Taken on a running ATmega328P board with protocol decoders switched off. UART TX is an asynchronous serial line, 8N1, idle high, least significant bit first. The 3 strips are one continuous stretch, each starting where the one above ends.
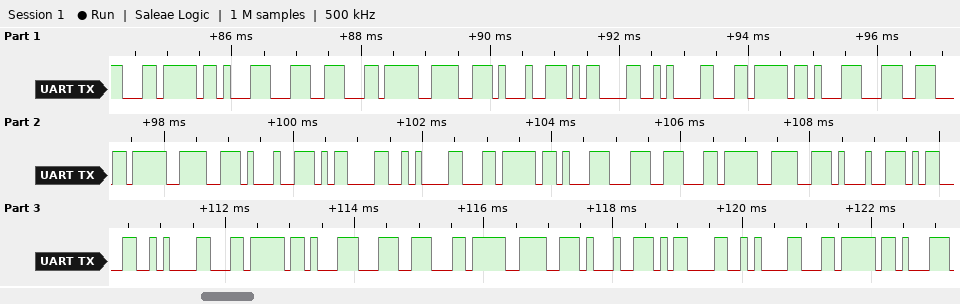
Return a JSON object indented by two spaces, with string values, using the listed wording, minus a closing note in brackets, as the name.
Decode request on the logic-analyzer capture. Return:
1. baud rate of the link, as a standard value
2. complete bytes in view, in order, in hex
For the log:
{
  "baud rate of the link, as a standard value": "9600 baud",
  "complete bytes in view, in order, in hex": "EC 8B 9C EC 9E 91 0D 0A EC 8B 9C EC 9E 91 0D 0A EC 8B 9C EC 9E 91 0D 0A EC 8B 9C EC 9E 91 0D 0A EC 8B"
}
